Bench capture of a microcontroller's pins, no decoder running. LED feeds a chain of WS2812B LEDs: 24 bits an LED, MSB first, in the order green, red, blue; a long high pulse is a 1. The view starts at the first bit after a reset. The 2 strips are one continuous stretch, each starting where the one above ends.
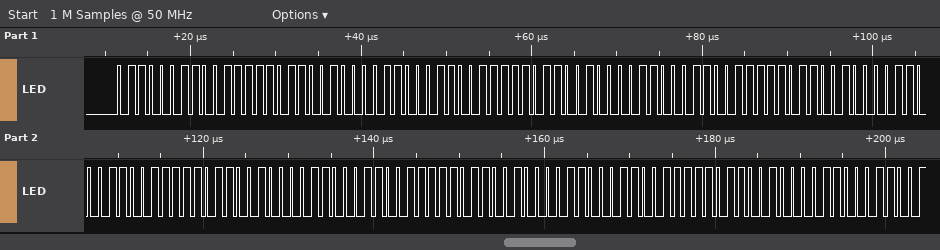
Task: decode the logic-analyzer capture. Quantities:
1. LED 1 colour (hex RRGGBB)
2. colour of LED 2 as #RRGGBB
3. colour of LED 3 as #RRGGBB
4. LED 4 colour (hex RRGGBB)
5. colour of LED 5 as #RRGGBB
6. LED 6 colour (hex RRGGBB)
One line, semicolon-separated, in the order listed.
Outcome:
#3E63C8; #3E63C8; #3E63C8; #3E63C8; #3E63C8; #3E63C8
